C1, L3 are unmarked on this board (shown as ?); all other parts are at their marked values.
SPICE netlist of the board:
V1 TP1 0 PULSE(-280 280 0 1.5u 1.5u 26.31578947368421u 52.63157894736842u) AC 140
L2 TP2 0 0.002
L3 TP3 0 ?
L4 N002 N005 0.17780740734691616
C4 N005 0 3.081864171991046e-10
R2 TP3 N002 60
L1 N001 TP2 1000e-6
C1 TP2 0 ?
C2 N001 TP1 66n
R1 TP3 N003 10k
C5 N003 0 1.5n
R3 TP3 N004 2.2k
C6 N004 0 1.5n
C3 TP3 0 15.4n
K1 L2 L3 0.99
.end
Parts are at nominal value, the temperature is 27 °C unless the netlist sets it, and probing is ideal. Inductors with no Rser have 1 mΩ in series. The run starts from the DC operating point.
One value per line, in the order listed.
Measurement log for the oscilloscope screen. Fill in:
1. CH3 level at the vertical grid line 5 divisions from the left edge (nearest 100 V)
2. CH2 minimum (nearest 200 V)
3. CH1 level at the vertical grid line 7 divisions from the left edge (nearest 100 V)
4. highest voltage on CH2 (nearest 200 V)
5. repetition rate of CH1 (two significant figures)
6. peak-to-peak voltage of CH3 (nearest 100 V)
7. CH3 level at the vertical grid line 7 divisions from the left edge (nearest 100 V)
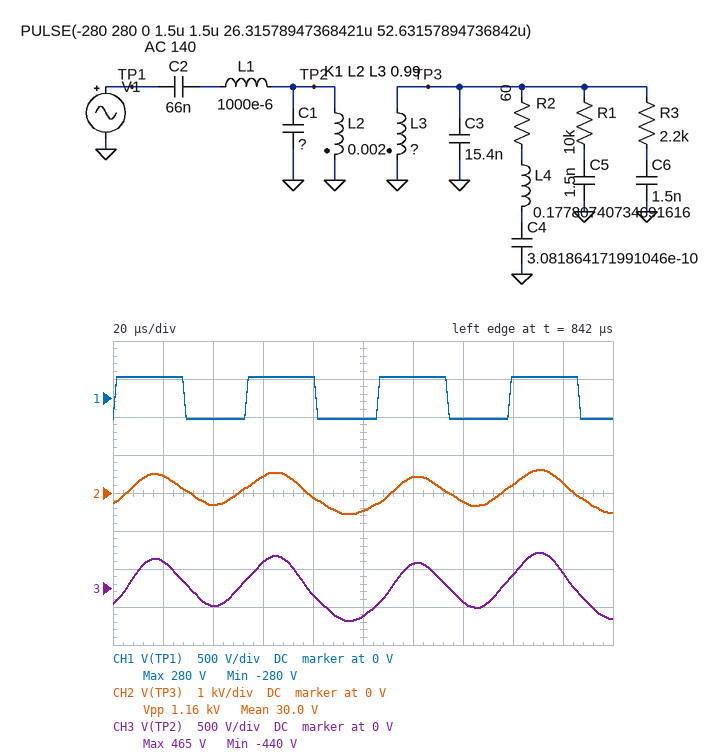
-400 V
-600 V
-300 V
600 V
19 kHz
900 V
-200 V
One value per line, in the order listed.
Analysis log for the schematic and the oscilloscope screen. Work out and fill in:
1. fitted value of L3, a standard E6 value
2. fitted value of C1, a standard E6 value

3.3 mH
47 nF
